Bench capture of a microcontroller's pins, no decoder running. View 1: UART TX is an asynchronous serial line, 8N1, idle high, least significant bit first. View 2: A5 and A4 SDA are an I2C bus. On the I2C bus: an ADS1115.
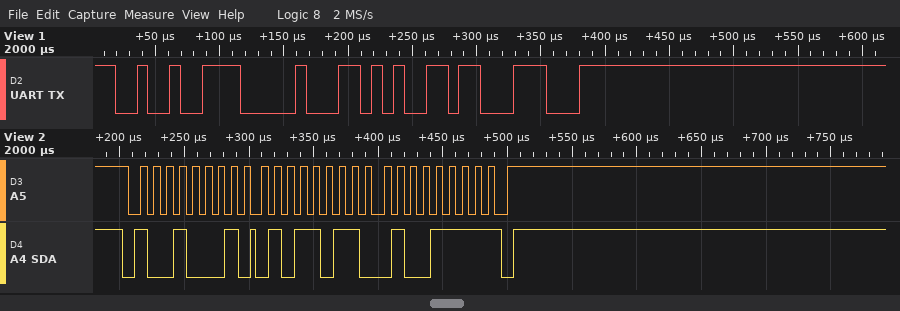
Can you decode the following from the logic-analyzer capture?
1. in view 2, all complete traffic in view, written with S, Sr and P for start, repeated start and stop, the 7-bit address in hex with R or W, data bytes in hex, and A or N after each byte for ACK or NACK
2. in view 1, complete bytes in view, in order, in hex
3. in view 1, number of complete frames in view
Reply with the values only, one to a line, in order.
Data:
S 48R A 5B A 4F N P
92 10 65 1C
4
